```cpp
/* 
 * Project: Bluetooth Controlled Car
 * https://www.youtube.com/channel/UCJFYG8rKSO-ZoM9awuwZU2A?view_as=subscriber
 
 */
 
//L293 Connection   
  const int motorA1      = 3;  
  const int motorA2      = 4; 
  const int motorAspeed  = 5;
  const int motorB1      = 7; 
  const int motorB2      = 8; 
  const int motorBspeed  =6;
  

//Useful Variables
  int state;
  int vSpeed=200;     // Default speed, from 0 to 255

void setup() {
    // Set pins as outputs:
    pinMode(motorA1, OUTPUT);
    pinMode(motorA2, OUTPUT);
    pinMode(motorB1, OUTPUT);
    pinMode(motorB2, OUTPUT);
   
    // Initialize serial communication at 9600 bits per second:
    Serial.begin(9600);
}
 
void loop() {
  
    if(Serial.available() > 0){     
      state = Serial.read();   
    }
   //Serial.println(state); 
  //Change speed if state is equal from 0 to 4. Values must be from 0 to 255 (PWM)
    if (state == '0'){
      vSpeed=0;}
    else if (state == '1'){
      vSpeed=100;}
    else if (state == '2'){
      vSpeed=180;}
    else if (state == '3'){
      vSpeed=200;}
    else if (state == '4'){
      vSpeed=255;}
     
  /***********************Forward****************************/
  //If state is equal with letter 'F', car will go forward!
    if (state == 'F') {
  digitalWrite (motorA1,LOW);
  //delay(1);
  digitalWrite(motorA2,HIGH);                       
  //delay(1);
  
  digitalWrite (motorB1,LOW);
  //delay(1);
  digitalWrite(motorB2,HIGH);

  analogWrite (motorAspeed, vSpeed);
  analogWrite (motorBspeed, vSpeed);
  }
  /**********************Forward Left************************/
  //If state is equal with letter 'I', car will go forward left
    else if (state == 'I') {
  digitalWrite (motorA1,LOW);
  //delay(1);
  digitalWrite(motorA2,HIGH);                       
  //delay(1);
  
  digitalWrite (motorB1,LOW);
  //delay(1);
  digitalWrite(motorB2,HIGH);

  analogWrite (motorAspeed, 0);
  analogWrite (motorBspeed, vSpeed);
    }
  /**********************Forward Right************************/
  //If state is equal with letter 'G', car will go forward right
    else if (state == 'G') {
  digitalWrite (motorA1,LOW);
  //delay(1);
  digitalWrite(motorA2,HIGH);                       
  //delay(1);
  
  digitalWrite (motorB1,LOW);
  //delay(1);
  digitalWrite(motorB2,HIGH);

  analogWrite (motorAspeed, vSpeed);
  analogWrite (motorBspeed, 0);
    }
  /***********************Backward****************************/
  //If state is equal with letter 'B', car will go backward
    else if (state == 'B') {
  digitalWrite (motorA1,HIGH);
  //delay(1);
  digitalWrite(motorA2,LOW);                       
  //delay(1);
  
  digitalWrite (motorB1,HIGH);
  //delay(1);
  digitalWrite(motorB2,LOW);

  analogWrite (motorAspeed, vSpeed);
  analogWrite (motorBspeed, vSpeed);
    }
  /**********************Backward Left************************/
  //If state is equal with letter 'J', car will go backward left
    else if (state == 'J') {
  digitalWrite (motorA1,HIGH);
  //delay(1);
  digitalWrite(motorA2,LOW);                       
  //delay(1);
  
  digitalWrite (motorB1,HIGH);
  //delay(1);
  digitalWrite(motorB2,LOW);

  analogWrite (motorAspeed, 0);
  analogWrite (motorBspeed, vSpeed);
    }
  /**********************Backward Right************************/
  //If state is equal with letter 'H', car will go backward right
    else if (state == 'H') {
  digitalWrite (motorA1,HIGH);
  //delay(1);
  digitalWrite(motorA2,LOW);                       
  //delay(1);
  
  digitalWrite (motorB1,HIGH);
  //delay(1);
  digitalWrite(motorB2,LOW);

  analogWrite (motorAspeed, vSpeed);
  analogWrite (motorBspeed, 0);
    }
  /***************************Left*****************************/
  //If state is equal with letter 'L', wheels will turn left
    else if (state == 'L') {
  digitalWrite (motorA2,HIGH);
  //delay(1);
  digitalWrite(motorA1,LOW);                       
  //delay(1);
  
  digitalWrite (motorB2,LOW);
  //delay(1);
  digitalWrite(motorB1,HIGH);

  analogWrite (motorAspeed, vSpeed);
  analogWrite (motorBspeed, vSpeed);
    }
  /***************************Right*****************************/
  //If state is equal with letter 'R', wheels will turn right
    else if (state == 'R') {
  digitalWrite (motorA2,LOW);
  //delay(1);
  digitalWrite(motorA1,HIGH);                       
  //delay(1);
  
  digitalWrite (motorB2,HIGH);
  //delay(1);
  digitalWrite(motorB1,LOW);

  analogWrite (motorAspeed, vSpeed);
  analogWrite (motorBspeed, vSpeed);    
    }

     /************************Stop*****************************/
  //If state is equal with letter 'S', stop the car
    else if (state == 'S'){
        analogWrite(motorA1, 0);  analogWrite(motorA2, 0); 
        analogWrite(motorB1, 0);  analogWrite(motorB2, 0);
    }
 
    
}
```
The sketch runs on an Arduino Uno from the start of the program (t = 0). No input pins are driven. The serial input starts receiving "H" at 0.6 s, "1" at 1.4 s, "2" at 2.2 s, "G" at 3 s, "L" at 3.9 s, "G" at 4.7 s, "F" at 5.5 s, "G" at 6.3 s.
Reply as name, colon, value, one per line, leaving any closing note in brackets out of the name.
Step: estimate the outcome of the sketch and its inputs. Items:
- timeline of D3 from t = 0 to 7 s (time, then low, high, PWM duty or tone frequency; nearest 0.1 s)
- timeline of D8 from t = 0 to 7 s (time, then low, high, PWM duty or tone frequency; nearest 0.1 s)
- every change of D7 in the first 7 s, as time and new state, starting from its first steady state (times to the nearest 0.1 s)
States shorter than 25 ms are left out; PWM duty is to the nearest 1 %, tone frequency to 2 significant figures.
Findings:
timeline of D3 from t = 0 to 7 s: 0 s low; 0.6 s high; 3 s low
timeline of D8 from t = 0 to 7 s: 0 s low; 3 s high; 3.9 s low; 4.7 s high
every change of D7 in the first 7 s, as time and new state, starting from its first steady state: 0 s low; 0.6 s high; 3 s low; 3.9 s high; 4.7 s low
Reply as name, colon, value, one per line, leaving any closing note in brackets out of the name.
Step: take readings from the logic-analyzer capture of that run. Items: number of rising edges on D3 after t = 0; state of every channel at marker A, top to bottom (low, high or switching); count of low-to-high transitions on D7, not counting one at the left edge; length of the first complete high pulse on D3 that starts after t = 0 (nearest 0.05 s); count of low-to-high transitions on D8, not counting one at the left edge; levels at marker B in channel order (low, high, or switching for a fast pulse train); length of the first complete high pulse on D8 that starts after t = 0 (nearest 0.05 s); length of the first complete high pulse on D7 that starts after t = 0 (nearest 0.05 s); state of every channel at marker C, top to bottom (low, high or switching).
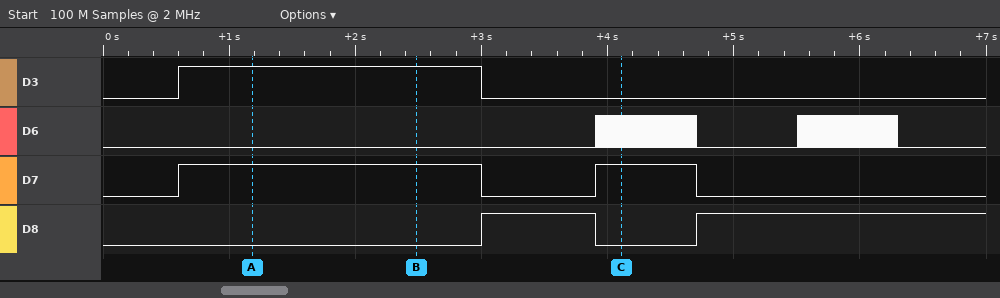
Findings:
number of rising edges on D3 after t = 0: 1
state of every channel at marker A, top to bottom: D3 high, D6 low, D7 high, D8 low
count of low-to-high transitions on D7, not counting one at the left edge: 2
length of the first complete high pulse on D3 that starts after t = 0: 2.40 s
count of low-to-high transitions on D8, not counting one at the left edge: 2
levels at marker B in channel order: D3 high, D6 low, D7 high, D8 low
length of the first complete high pulse on D8 that starts after t = 0: 0.90 s
length of the first complete high pulse on D7 that starts after t = 0: 2.40 s
state of every channel at marker C, top to bottom: D3 low, D6 switching, D7 high, D8 low
